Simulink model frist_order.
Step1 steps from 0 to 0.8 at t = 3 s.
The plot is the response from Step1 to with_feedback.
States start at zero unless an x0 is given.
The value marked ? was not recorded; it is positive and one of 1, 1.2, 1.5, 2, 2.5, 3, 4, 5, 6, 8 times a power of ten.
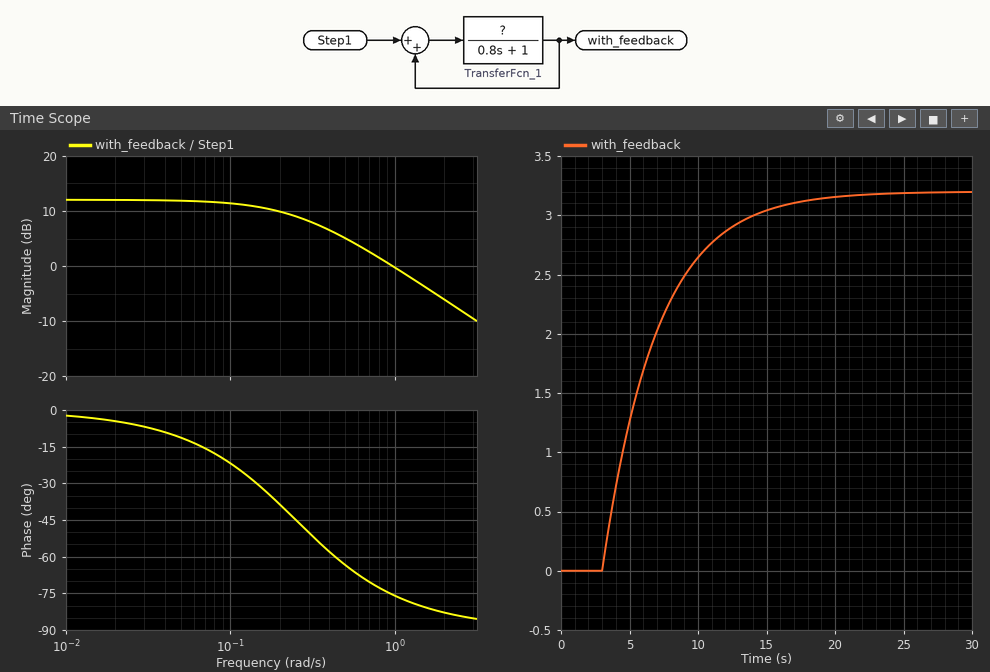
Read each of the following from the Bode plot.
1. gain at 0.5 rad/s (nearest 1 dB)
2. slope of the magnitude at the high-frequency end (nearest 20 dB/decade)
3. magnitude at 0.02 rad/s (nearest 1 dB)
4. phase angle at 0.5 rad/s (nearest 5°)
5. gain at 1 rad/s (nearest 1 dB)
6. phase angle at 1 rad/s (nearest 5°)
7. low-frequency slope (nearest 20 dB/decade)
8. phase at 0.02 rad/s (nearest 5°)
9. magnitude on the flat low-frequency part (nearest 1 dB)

5 dB
-20 dB/decade
12 dB
-65°
0 dB
-75°
0 dB/decade
-5°
12 dB
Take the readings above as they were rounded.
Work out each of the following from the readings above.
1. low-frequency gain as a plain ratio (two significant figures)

4.0
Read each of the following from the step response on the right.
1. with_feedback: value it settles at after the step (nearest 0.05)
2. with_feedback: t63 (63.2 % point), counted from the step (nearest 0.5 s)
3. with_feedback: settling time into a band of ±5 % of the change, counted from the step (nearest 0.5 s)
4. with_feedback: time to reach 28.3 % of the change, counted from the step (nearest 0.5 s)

3.20
4.0 s
12.0 s
1.5 s
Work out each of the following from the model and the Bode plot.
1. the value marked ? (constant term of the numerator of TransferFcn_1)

0.8
